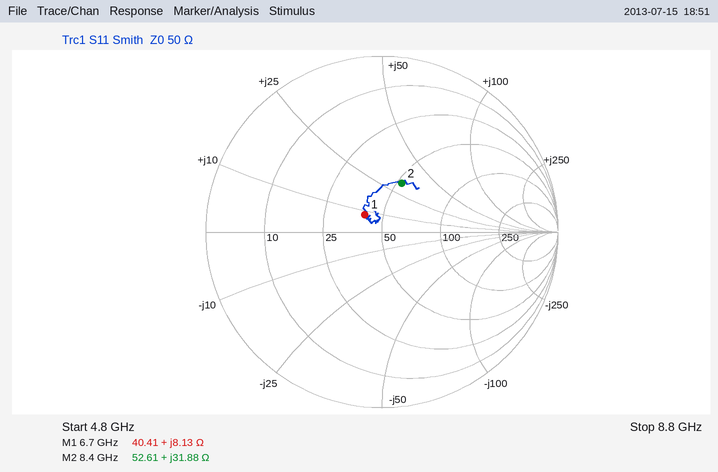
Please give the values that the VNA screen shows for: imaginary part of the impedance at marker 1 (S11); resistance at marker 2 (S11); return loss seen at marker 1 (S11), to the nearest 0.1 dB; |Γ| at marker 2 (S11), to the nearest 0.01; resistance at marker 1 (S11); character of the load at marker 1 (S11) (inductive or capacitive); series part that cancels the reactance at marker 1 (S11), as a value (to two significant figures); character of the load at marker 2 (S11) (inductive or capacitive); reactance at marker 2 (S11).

+8.13 Ω
52.61 Ω
17.2 dB
0.30
40.41 Ω
inductive
2.9 pF
inductive
+31.88 Ω
